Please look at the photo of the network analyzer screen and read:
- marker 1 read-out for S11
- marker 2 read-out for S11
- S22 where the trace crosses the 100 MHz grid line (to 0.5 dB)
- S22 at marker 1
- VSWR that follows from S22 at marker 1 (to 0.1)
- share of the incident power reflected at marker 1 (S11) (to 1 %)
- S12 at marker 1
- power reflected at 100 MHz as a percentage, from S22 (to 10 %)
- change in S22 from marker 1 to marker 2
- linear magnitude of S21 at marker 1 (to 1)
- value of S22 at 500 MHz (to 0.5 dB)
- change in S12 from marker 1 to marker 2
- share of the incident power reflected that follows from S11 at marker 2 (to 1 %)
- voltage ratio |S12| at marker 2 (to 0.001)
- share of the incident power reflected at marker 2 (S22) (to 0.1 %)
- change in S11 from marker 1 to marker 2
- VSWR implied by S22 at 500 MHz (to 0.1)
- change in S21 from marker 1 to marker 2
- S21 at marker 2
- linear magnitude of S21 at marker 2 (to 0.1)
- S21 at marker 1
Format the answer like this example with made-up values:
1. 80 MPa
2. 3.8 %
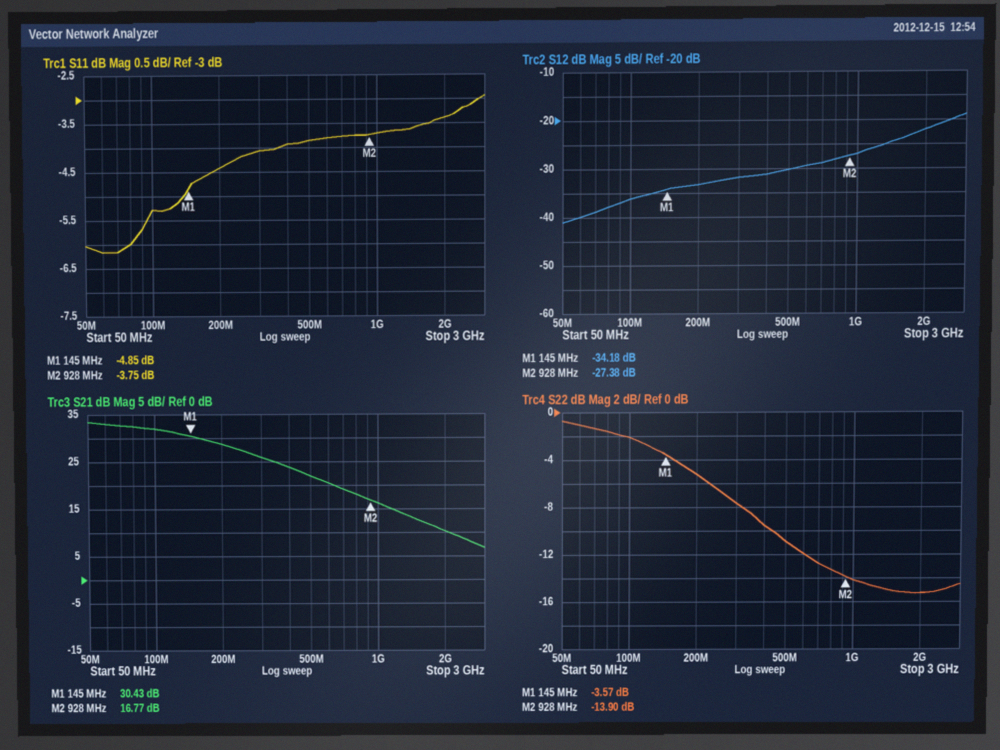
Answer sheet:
1. -4.85 dB
2. -3.75 dB
3. -2.0 dB
4. -3.57 dB
5. 4.9
6. 33 %
7. -34.18 dB
8. 60 %
9. -10.33 dB
10. 33
11. -11.0 dB
12. 6.80 dB
13. 42 %
14. 0.043
15. 4.1 %
16. 1.10 dB
17. 1.8
18. -13.66 dB
19. 16.77 dB
20. 6.9
21. 30.43 dB
